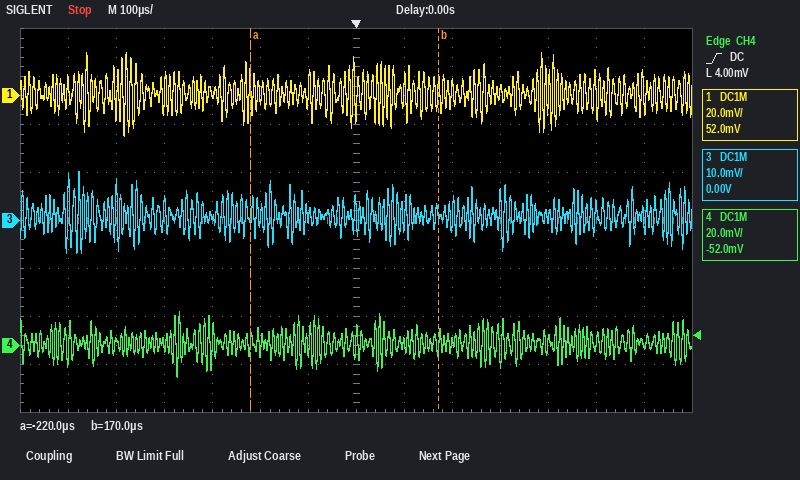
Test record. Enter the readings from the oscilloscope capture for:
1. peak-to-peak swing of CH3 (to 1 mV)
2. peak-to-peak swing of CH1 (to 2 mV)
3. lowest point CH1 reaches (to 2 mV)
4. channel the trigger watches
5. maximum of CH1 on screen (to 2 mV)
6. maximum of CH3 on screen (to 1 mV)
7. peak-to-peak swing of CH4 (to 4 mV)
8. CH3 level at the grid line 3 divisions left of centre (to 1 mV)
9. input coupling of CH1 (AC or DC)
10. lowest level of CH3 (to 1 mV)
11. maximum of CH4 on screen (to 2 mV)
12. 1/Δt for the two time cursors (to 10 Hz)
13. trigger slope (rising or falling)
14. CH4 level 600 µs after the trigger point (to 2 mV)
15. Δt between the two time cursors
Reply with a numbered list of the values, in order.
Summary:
1. 17 mV
2. 34 mV
3. -16 mV
4. CH4
5. 18 mV
6. 10 mV
7. 28 mV
8. 1 mV
9. DC
10. -7 mV
11. 14 mV
12. 2.56 kHz
13. rising
14. 0 mV
15. 390 µs
